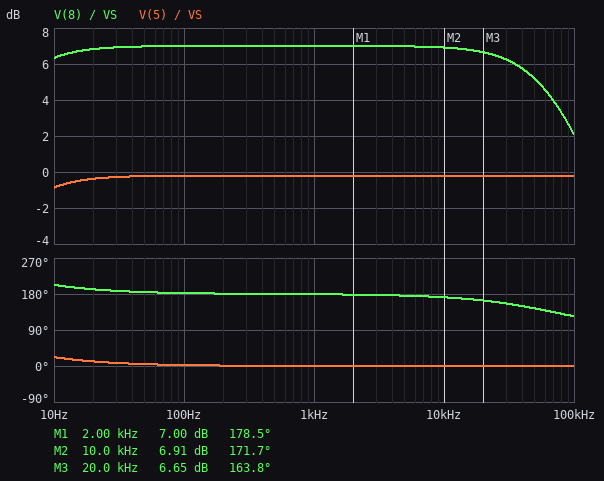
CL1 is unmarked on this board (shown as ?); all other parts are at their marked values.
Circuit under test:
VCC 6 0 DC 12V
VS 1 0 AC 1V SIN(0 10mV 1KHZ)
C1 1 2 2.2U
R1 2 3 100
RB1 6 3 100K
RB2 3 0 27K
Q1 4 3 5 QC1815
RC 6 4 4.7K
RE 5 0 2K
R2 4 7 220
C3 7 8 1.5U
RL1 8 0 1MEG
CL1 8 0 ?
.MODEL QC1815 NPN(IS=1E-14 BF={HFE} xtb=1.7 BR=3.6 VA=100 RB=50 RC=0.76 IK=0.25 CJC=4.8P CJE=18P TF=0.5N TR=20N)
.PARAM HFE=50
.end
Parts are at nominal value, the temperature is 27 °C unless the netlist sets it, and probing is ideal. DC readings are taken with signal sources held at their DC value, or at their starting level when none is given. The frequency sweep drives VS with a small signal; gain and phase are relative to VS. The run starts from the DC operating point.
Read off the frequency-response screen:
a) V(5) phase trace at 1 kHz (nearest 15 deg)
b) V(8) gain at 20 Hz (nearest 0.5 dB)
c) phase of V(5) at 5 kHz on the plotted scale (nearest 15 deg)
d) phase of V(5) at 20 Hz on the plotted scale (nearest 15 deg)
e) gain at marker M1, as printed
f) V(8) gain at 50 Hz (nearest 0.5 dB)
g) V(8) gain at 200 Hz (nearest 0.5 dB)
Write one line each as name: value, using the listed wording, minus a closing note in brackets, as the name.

V(5) phase trace at 1 kHz: 0 deg
V(8) gain at 20 Hz: 7.0 dB
phase of V(5) at 5 kHz on the plotted scale: 0 deg
phase of V(5) at 20 Hz on the plotted scale: 15 deg
gain at marker M1, as printed: 7.00 dB
V(8) gain at 50 Hz: 7.0 dB
V(8) gain at 200 Hz: 7.0 dB
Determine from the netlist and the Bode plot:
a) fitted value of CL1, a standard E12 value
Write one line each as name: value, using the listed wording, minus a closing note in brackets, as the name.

fitted value of CL1, a standard E12 value: 470 pF
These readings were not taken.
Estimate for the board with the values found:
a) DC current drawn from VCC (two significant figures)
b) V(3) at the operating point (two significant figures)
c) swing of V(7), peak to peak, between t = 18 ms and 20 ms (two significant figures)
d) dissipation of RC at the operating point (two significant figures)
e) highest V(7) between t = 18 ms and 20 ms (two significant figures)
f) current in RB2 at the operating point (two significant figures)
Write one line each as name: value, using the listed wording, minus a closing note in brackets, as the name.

DC current drawn from VCC: 880 µA
V(3) at the operating point: 2.2 V
swing of V(7), peak to peak, between t = 18 ms and 20 ms: 45 mV
dissipation of RC at the operating point: 2.9 mW
highest V(7) between t = 18 ms and 20 ms: 8.4 V
current in RB2 at the operating point: 83 µA
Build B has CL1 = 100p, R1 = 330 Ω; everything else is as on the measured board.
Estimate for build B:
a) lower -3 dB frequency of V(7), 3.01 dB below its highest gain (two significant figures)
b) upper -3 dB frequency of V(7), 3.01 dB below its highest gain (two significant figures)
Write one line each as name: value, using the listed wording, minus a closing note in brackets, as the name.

lower -3 dB frequency of V(7), 3.01 dB below its highest gain: 4.0 Hz
upper -3 dB frequency of V(7), 3.01 dB below its highest gain: 320 kHz
